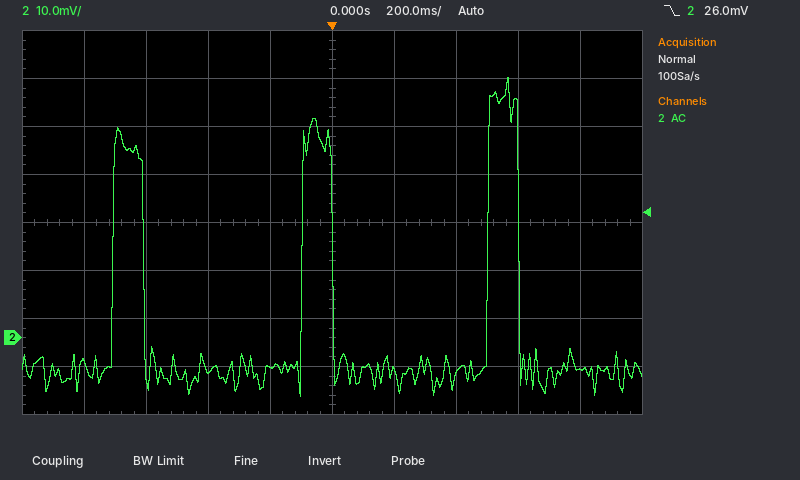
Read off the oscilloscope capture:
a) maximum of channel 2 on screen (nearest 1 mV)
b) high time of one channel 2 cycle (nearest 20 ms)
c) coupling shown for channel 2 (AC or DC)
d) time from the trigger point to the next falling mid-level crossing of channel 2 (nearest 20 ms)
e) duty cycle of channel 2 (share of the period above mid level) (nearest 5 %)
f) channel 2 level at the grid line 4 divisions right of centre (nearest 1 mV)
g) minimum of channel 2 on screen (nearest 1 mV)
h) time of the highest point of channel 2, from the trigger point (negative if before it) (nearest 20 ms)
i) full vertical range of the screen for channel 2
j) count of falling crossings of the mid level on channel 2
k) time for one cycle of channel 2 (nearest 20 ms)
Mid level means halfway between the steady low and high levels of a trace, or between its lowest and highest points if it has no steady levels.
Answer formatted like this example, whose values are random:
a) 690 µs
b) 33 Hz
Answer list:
a) 54 mV
b) 100 ms
c) AC
d) 600 ms
e) 15 %
f) -7 mV
g) -12 mV
h) +560 ms
i) 80 mV
j) 3
k) 600 ms
